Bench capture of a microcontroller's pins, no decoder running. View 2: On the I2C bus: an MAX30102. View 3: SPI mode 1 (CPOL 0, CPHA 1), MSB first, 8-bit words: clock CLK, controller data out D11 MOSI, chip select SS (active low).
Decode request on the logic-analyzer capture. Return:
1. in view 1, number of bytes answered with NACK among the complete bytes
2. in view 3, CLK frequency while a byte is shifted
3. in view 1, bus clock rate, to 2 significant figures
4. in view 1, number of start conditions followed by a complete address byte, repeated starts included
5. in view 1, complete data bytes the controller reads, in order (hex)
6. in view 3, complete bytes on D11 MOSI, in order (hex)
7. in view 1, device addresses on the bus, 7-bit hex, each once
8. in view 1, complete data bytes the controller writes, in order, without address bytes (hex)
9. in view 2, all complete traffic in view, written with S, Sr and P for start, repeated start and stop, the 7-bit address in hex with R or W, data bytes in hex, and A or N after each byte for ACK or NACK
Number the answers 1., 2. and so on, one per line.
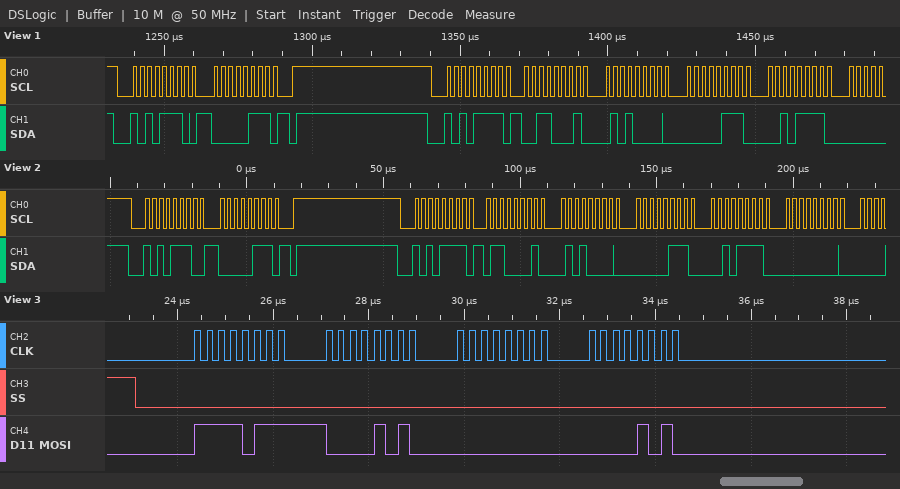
1. 0
2. 4 MHz
3. 400 kHz
4. 2
5. 31 50 07 2F
6. F7 0A 00 0A
7. 0x57
8. 07
9. S 57W A 07 A P S 57R A 61 A 50 A 07 A 2F A 00 A
